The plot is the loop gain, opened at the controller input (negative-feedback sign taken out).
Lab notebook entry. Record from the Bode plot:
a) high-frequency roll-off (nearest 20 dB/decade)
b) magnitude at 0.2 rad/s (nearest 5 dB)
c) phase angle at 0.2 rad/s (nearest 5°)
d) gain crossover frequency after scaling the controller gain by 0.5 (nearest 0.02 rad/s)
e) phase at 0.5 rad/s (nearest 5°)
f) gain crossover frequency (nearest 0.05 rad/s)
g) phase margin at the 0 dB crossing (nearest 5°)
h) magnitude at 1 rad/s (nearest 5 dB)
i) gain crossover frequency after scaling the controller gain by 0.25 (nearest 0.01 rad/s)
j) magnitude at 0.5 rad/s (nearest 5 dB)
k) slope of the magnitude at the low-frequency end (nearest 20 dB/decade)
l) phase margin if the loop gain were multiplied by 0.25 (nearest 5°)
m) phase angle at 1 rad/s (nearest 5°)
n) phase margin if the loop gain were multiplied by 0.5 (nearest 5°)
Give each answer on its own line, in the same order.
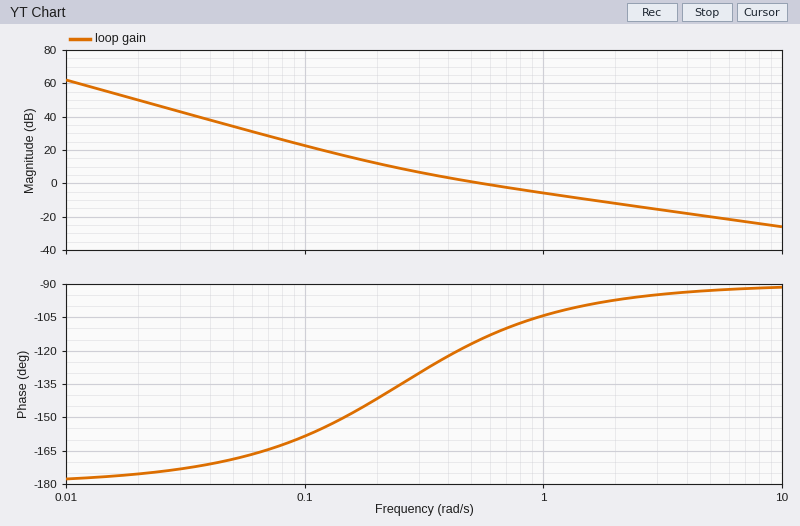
-20 dB/decade
10 dB
-140°
0.32 rad/s
-115°
0.55 rad/s
65°
-5 dB
0.20 rad/s
0 dB
-40 dB/decade
40°
-105°
50°
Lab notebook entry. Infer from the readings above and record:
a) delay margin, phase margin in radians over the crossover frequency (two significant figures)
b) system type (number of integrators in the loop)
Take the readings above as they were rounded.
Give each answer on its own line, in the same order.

2.1 s
2
